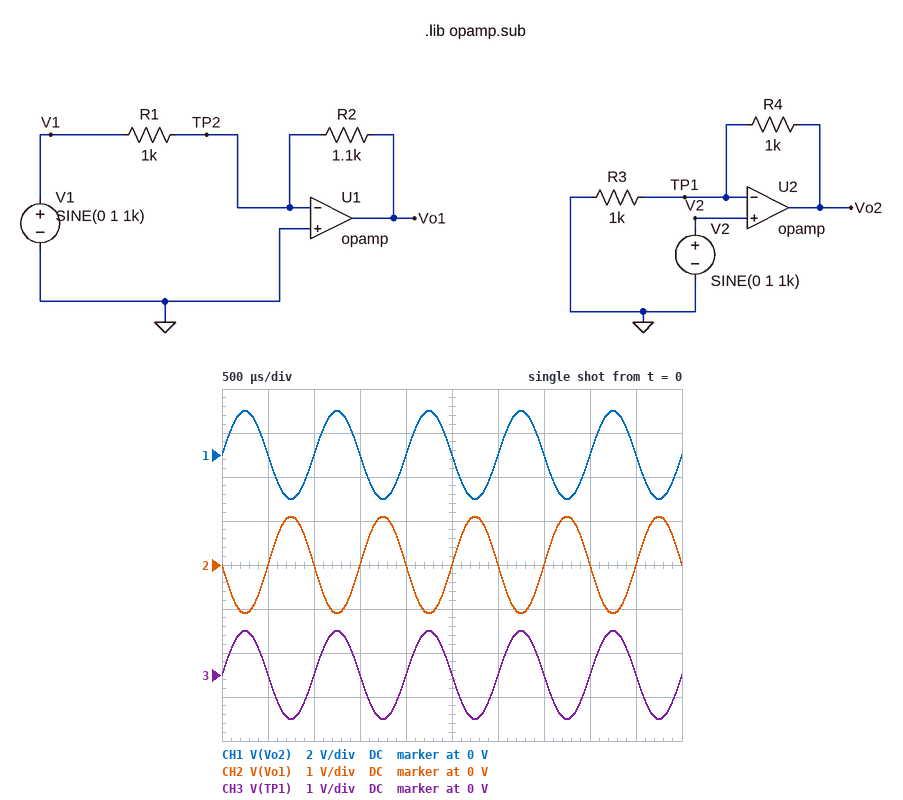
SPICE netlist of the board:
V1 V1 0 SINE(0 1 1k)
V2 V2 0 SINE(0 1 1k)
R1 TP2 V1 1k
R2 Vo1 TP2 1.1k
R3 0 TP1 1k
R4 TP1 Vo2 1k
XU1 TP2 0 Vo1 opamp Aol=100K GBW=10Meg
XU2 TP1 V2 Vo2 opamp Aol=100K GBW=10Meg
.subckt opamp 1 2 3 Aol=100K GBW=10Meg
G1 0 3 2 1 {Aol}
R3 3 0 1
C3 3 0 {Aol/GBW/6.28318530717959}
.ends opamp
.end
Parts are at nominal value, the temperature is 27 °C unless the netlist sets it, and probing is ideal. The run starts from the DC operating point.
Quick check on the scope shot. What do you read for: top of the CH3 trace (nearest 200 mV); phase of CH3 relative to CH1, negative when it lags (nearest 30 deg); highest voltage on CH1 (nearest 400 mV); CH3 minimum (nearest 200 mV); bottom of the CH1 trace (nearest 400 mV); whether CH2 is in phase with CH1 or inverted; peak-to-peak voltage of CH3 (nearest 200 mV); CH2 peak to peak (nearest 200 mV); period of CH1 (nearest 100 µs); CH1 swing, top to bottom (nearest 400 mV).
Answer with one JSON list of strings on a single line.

["1.0 V", "0 deg", "2.0 V", "-1.0 V", "-2.0 V", "inverted", "2.0 V", "2.2 V", "1.0 ms", "4.0 V"]
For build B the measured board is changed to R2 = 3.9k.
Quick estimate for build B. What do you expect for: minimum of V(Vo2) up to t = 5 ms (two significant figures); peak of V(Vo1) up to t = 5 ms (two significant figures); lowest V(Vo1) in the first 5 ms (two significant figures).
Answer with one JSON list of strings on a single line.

["-2.0 V", "3.9 V", "-3.9 V"]
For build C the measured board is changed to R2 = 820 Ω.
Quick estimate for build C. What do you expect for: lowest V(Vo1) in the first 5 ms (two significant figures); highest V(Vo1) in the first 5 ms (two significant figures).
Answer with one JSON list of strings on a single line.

["-820 mV", "820 mV"]
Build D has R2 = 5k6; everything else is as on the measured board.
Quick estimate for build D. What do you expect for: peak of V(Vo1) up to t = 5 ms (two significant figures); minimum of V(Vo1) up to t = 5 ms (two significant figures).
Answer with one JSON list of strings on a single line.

["5.6 V", "-5.6 V"]
